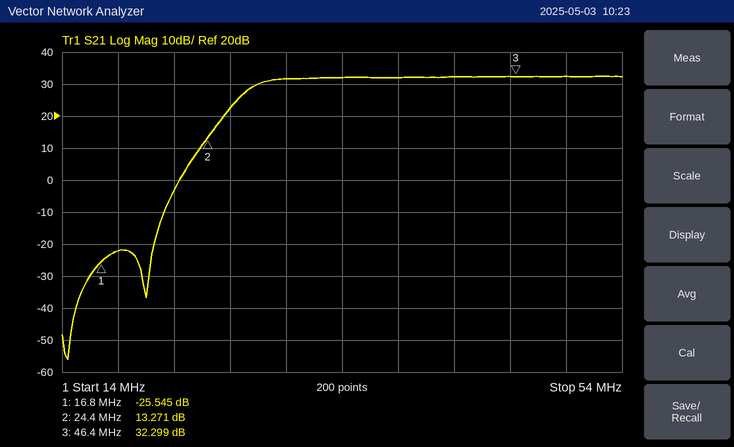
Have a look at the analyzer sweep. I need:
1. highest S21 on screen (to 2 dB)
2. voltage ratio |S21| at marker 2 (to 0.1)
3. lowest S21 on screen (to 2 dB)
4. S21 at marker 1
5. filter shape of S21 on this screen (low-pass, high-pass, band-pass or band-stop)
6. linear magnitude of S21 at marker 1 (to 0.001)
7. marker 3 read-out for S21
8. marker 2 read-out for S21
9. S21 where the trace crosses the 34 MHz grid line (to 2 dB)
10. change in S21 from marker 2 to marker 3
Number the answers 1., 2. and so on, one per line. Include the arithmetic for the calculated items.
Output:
1. 32 dB
2. 10^(13.271/20) ≈ 4.6
3. -56 dB
4. -25.545 dB
5. high-pass
6. 10^(-25.545/20) ≈ 0.053
7. 32.299 dB
8. 13.271 dB
9. 32 dB
10. 32.299 − (13.271) = 19.028 dB
